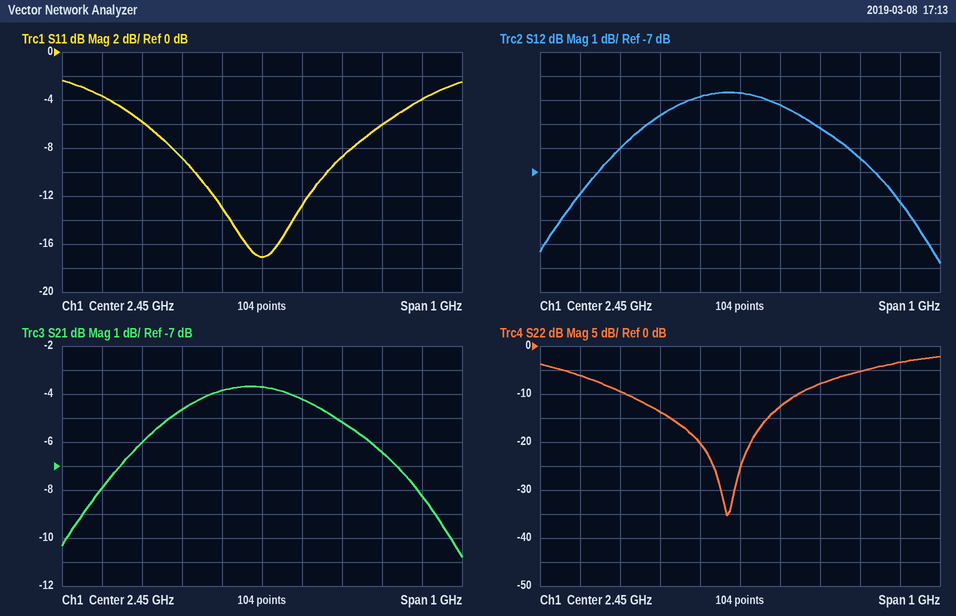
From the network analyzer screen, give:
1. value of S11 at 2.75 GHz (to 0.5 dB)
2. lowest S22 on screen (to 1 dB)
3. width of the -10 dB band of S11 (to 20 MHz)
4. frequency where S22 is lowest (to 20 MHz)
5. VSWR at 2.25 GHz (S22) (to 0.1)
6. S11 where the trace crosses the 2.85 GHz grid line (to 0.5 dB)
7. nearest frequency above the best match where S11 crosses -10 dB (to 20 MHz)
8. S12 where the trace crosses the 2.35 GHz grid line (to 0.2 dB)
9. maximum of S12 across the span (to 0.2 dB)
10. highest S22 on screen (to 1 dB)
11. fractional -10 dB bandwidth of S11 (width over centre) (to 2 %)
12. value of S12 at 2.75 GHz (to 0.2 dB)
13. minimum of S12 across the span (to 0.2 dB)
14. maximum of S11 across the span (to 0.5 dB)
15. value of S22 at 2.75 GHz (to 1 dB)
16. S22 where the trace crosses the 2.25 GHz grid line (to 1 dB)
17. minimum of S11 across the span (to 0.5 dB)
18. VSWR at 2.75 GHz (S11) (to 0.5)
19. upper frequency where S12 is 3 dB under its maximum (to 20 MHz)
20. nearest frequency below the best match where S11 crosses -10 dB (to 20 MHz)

-6.0 dB
-35 dB
340 MHz
2.42 GHz
1.5
-4.0 dB
2.62 GHz
-3.8 dB
-3.6 dB
-2 dB
14 %
-6.4 dB
-10.8 dB
-2.5 dB
-5 dB
-14 dB
-17.0 dB
3.0
2.76 GHz
2.28 GHz
